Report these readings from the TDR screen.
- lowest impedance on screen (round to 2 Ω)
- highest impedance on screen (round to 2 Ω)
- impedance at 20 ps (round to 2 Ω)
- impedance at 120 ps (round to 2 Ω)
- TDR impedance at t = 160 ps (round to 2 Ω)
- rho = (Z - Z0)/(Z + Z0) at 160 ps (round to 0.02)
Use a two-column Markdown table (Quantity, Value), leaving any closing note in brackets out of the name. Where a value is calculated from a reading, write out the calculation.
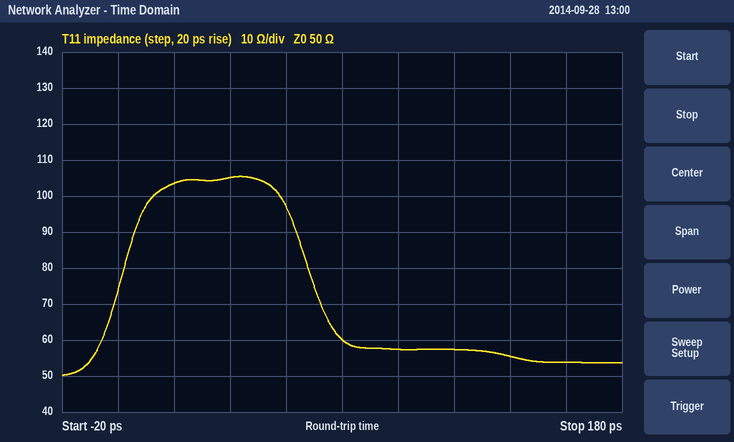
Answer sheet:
| Quantity | Value |
|---|---|
| lowest impedance on screen | 50 Ω |
| highest impedance on screen | 106 Ω |
| impedance at 20 ps | 104 Ω |
| impedance at 120 ps | 58 Ω |
| TDR impedance at t = 160 ps | 54 Ω |
| rho = (Z - Z0)/(Z + Z0) at 160 ps | (54 − 50)/(54 + 50) ≈ +0.04 |
